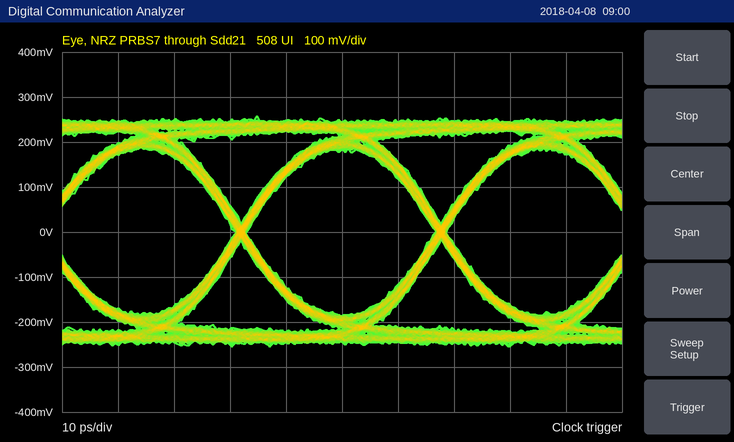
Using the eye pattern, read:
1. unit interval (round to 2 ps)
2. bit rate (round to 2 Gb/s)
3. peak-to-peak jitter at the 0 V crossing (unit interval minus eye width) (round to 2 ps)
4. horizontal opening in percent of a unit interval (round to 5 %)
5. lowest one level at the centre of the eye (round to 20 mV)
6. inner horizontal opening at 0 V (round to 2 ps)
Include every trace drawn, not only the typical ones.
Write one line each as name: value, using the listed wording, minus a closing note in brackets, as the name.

unit interval: 36 ps
bit rate: 28 Gb/s
peak-to-peak jitter at the 0 V crossing (unit interval minus eye width): 2 ps
horizontal opening in percent of a unit interval: 95 %
lowest one level at the centre of the eye: 180 mV
inner horizontal opening at 0 V: 34 ps
